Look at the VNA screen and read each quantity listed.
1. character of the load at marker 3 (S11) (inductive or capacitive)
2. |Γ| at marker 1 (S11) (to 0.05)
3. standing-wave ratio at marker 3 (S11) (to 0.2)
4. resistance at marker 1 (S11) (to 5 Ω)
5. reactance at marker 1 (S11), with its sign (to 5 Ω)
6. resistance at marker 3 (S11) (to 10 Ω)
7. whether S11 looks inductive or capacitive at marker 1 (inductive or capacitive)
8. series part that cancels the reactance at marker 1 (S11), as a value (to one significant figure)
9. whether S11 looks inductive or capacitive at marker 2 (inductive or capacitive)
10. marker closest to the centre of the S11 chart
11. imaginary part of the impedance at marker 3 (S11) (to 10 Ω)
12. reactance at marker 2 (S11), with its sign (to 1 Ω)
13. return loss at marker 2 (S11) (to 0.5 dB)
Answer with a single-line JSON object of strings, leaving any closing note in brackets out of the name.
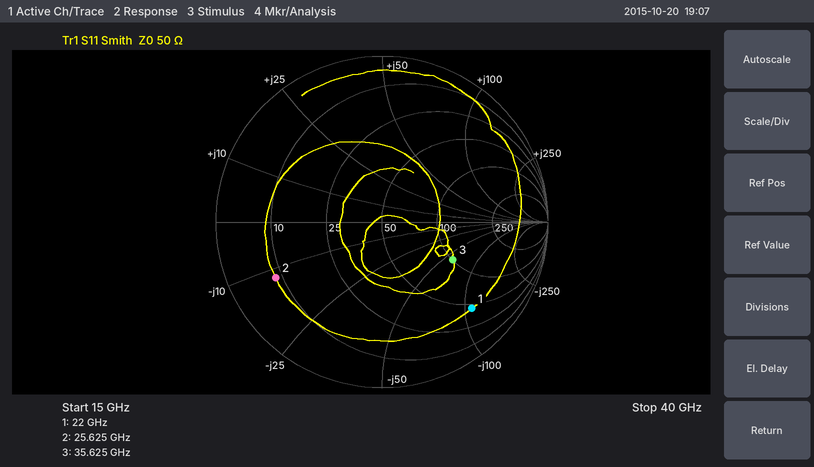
{"character of the load at marker 3 (S11)": "capacitive", "|Γ| at marker 1 (S11)": "0.75", "standing-wave ratio at marker 3 (S11)": "2.8", "resistance at marker 1 (S11)": "45 Ω", "reactance at marker 1 (S11), with its sign": "-110 Ω", "resistance at marker 3 (S11)": "100 Ω", "whether S11 looks inductive or capacitive at marker 1": "capacitive", "series part that cancels the reactance at marker 1 (S11), as a value": "800 pH", "whether S11 looks inductive or capacitive at marker 2": "capacitive", "marker closest to the centre of the S11 chart": "marker 3", "imaginary part of the impedance at marker 3 (S11)": "-60 Ω", "reactance at marker 2 (S11), with its sign": "-12 Ω", "return loss at marker 2 (S11)": "3.0 dB"}
